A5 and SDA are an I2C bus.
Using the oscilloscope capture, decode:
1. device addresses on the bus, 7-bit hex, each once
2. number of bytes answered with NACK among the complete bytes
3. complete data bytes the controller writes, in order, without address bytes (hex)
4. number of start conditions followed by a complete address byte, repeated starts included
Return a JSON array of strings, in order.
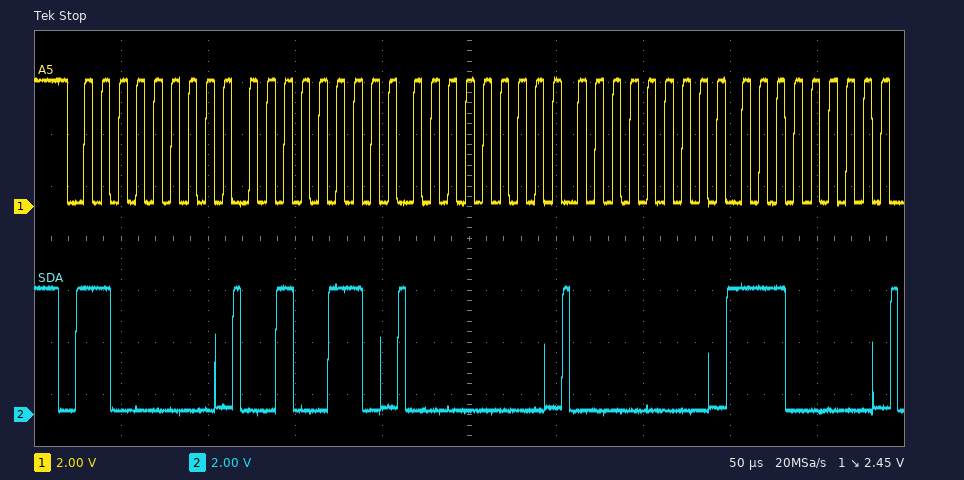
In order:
["0x60", "0", "26 00 00 E0", "1"]
